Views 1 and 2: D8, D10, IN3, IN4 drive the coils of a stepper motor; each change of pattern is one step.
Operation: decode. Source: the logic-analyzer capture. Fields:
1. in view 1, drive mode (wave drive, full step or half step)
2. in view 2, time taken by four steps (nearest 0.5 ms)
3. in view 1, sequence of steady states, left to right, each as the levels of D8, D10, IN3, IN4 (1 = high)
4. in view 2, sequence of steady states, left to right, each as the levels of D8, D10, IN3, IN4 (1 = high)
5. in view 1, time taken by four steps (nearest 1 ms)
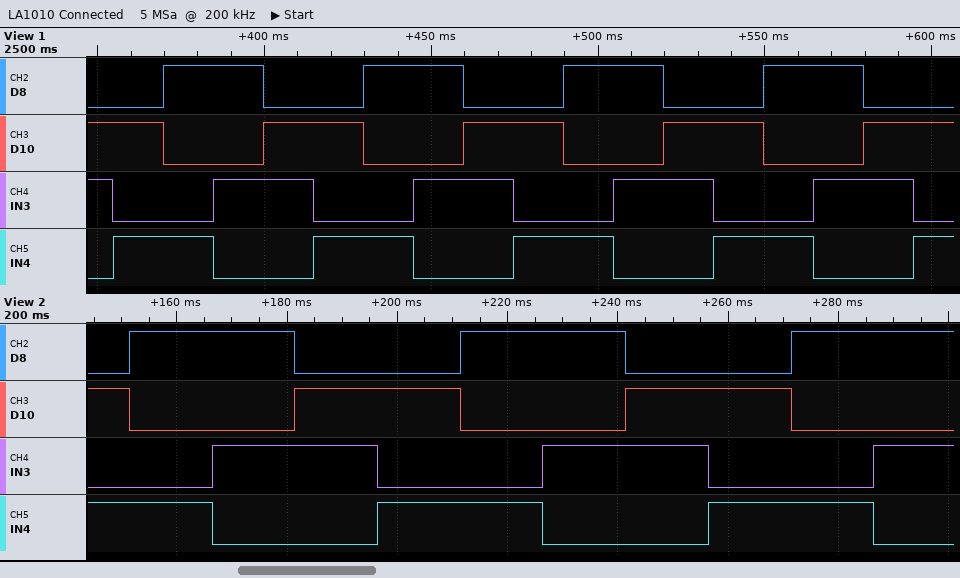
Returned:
full step
60.0 ms
0110 0101 1001 1010 0110 0101 1001 1010 0110 0101 1001 1010 0110 0101 1001 1010 0110 0101
0101 1001 1010 0110 0101 1001 1010 0110 0101 1001 1010
60 ms
